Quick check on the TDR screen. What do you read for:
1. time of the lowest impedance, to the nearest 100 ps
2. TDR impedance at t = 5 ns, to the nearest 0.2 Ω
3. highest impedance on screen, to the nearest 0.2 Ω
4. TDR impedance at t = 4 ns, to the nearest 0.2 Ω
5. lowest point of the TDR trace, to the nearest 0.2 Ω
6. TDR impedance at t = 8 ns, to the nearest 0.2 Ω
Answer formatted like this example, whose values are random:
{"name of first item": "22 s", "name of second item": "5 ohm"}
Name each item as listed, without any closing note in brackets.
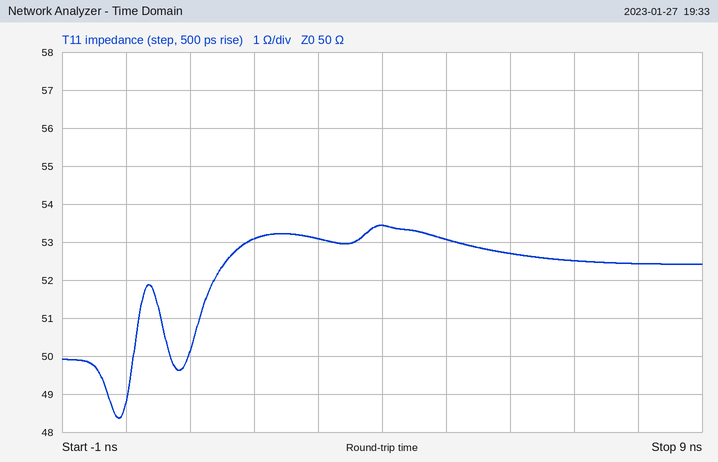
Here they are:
{"time of the lowest impedance, to the nearest 100 ps": "-100 ps", "TDR impedance at t = 5 ns, to the nearest 0.2 Ω": "53.0 Ω", "highest impedance on screen, to the nearest 0.2 Ω": "53.4 Ω", "TDR impedance at t = 4 ns, to the nearest 0.2 Ω": "53.4 Ω", "lowest point of the TDR trace, to the nearest 0.2 Ω": "48.4 Ω", "TDR impedance at t = 8 ns, to the nearest 0.2 Ω": "52.4 Ω"}
